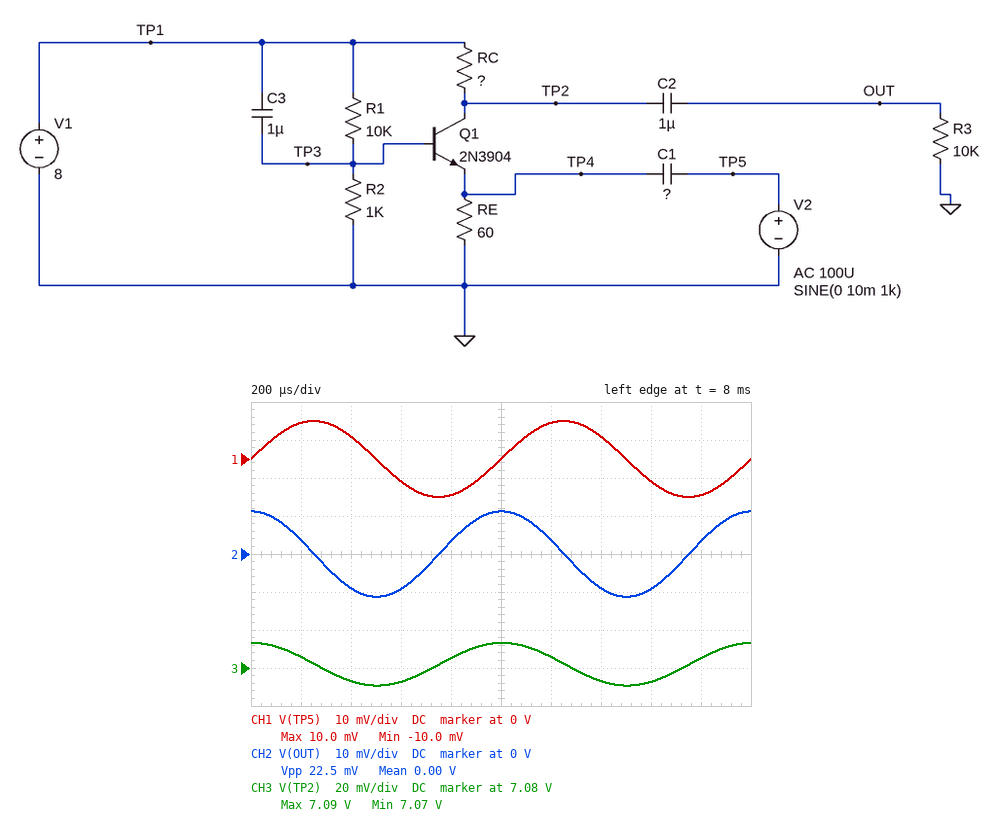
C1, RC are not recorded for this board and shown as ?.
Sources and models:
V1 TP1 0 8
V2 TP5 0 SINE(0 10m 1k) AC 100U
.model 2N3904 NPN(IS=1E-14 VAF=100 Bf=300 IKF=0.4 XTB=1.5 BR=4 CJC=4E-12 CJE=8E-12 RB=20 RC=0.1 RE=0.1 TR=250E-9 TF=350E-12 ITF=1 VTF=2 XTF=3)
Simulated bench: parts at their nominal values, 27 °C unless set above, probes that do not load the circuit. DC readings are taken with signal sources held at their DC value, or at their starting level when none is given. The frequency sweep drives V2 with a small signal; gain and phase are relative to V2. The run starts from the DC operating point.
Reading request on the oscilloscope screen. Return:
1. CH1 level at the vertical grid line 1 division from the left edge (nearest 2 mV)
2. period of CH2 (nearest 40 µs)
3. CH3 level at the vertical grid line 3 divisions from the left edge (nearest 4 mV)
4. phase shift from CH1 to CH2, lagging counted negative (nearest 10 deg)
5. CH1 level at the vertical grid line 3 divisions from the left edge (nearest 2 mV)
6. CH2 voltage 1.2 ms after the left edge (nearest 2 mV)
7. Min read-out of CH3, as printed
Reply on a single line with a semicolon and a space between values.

10 mV; 1.00 ms; 7.072 V; 90 deg; -6 mV; 4 mV; 7.07 V
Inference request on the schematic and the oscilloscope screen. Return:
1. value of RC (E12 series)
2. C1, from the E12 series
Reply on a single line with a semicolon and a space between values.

820 Ω; 330 nF
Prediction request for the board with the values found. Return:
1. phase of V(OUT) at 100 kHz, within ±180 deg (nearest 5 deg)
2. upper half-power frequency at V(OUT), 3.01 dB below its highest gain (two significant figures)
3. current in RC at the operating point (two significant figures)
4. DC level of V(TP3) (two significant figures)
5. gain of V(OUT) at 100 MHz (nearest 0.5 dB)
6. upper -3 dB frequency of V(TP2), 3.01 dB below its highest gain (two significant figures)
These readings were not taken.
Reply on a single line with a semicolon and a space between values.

15 deg; 53 MHz; 1.1 mA; 720 mV; 23.5 dB; 53 MHz
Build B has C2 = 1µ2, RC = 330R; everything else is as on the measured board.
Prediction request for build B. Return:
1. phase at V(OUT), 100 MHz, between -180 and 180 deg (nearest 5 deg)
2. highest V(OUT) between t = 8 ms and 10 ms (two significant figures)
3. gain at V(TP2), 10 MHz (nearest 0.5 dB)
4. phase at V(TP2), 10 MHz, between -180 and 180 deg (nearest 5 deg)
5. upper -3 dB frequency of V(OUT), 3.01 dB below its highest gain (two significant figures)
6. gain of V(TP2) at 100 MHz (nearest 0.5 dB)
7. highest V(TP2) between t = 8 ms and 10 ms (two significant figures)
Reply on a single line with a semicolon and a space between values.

-50 deg; 4.7 mV; 22.5 dB; -5 deg; 100 MHz; 20.0 dB; 7.6 V
